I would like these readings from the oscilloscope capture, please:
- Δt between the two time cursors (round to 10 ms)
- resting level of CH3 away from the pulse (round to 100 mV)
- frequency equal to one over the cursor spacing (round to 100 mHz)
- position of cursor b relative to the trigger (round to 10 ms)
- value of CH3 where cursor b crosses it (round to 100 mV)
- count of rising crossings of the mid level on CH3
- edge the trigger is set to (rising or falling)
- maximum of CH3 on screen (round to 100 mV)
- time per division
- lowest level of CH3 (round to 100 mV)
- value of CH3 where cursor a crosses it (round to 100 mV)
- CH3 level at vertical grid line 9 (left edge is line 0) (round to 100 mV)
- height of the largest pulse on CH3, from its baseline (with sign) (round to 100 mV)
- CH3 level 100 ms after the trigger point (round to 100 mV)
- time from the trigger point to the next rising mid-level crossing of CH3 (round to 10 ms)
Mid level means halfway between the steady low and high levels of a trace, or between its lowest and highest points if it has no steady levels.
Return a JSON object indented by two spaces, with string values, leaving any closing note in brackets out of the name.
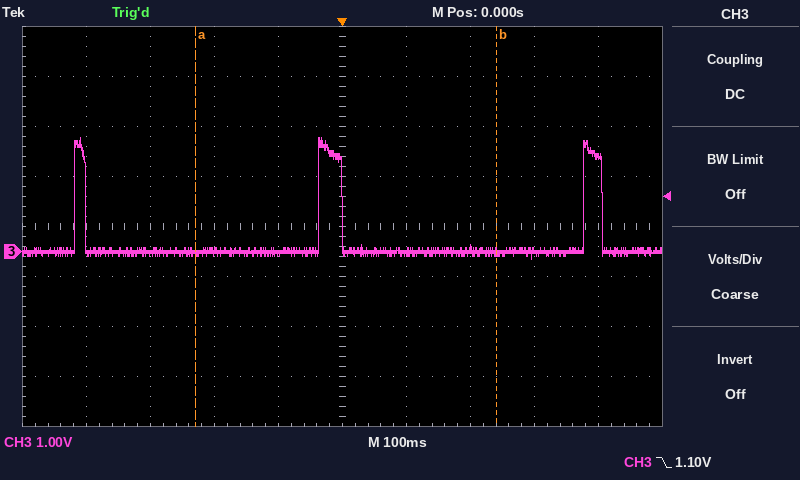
{
  "Δt between the two time cursors": "470 ms",
  "resting level of CH3 away from the pulse": "0.0 V",
  "frequency equal to one over the cursor spacing": "2.1 Hz",
  "position of cursor b relative to the trigger": "+240 ms",
  "value of CH3 where cursor b crosses it": "0.0 V",
  "count of rising crossings of the mid level on CH3": "3",
  "edge the trigger is set to": "falling",
  "maximum of CH3 on screen": "2.3 V",
  "time per division": "100 ms",
  "lowest level of CH3": "-200 mV",
  "value of CH3 where cursor a crosses it": "0.0 V",
  "CH3 level at vertical grid line 9 (left edge is line 0)": "1.9 V",
  "height of the largest pulse on CH3, from its baseline (with sign)": "+2.3 V",
  "CH3 level 100 ms after the trigger point": "0.0 V",
  "time from the trigger point to the next rising mid-level crossing of CH3": "380 ms"
}
